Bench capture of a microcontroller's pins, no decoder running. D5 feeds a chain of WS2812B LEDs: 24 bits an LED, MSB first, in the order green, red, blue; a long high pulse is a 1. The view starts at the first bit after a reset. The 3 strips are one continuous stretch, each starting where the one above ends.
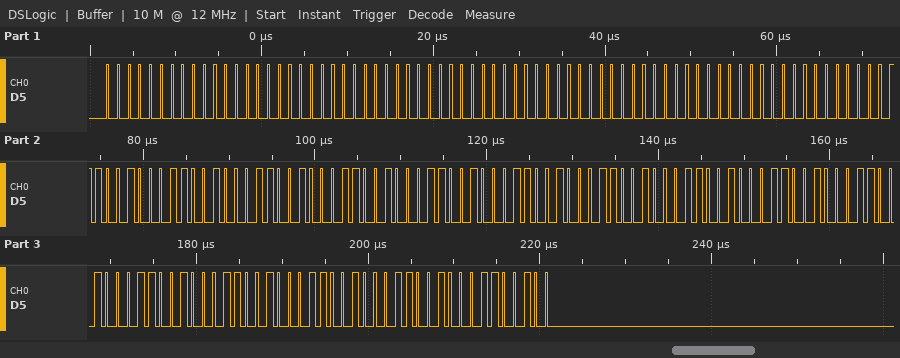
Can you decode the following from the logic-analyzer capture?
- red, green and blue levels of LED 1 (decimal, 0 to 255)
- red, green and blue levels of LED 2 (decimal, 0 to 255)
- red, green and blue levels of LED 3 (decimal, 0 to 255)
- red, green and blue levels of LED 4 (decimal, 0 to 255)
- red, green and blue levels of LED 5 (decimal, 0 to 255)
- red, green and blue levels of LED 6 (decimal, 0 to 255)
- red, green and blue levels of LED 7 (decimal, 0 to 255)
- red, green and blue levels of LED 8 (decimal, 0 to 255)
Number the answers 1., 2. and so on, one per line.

1. 0, 0, 0
2. 0, 0, 0
3. 0, 0, 0
4. 100, 100, 100
5. 100, 100, 100
6. 100, 100, 100
7. 100, 100, 100
8. 100, 100, 100
